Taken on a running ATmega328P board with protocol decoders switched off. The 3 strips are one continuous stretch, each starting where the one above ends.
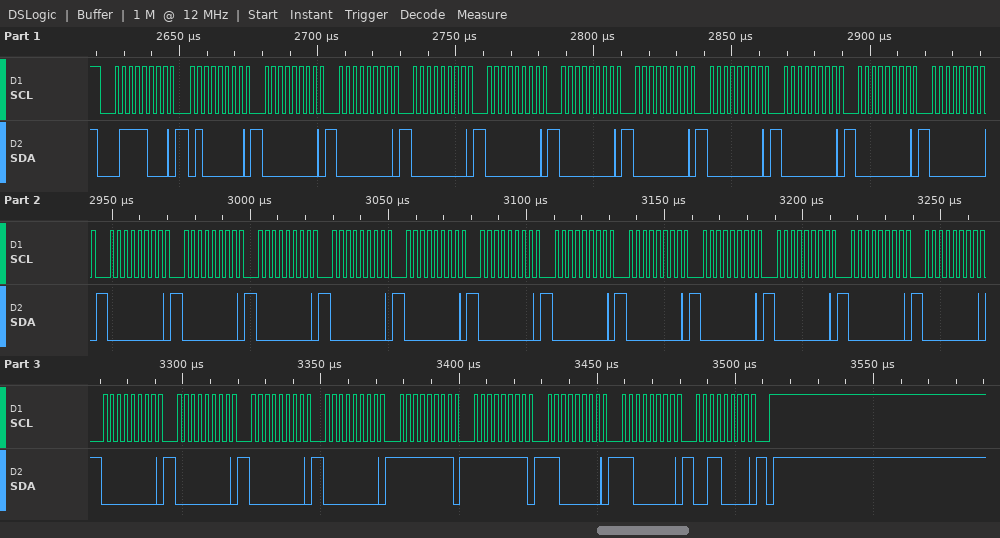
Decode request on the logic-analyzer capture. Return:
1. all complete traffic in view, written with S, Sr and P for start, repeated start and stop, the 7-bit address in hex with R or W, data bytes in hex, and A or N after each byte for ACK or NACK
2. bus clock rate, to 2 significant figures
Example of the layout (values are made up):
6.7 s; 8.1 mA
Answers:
S 3CW A 40 A 00 A 00 A 00 A 00 A 00 A 00 A 00 A 00 A 00 A 00 A 00 A 00 A 00 A 00 A 00 A 00 A 00 A 00 A 00 A 00 A 00 A 00 A 00 A 00 A 00 A 00 A FF A FF A C0 A C0 A 30 A P; 400 kHz
